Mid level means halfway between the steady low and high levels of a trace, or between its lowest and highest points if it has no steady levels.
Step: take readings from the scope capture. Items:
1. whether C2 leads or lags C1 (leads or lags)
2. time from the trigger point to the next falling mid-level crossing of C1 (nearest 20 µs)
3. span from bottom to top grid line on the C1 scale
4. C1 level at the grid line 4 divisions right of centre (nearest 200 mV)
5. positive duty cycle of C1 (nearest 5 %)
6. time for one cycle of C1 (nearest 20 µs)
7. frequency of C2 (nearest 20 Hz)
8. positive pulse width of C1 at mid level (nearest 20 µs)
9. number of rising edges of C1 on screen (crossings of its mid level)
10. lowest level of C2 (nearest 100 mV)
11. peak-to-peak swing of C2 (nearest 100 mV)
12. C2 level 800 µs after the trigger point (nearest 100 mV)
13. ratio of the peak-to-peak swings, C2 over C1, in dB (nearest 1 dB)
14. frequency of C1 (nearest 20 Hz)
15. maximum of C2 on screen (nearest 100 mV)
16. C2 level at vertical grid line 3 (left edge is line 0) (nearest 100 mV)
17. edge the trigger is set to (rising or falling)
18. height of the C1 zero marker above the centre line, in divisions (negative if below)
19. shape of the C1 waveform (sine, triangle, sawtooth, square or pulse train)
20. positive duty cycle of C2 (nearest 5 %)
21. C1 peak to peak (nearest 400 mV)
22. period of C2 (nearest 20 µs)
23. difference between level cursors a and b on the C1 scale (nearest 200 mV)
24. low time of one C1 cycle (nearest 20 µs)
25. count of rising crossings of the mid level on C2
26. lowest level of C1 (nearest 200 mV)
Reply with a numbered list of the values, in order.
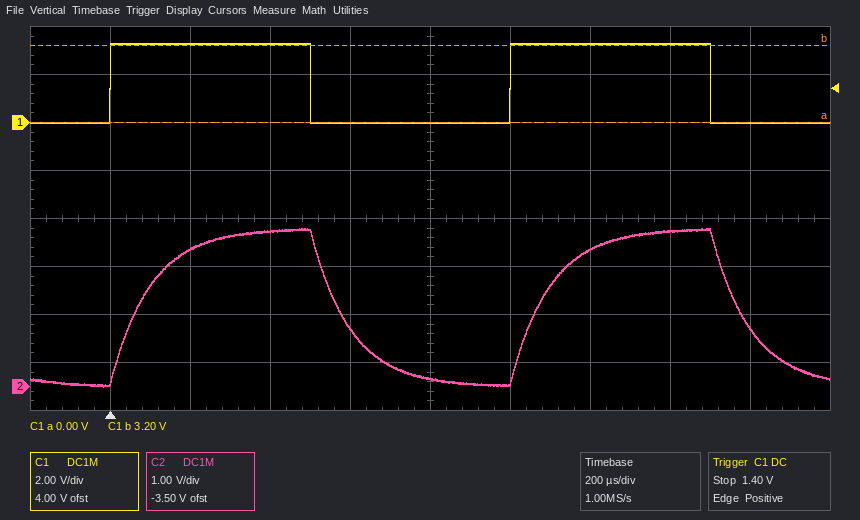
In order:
1. lags
2. 500 µs
3. 16 V
4. 0.0 V
5. 50 %
6. 1.00 ms
7. 1.00 kHz
8. 500 µs
9. 2
10. 0.0 V
11. 3.3 V
12. 200 mV
13. 0 dB
14. 1.00 kHz
15. 3.3 V
16. 3.2 V
17. rising
18. +2.0 div
19. square
20. 50 %
21. 3.2 V
22. 1.00 ms
23. 3.2 V
24. 500 µs
25. 2
26. 0.0 V
